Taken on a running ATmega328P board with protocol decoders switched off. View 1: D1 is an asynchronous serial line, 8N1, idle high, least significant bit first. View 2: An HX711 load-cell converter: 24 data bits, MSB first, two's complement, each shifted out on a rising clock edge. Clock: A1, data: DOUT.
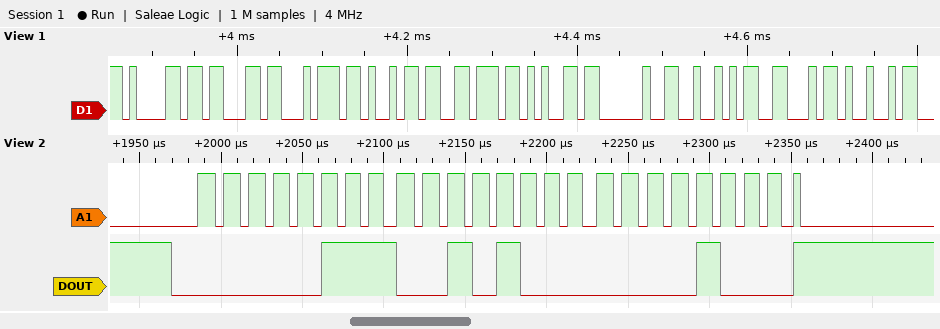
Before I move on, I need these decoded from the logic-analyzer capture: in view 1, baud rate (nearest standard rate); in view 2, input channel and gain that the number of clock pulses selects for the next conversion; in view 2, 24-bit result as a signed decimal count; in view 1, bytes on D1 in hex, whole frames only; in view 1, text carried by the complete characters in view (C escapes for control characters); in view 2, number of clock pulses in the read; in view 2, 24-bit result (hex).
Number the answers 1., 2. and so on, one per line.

1. 115200 baud
2. channel A, gain 128
3. 469000
4. 61 63 74 69 76 65 20 52 46 49
5. "active RFI"
6. 25
7. 0x072808
